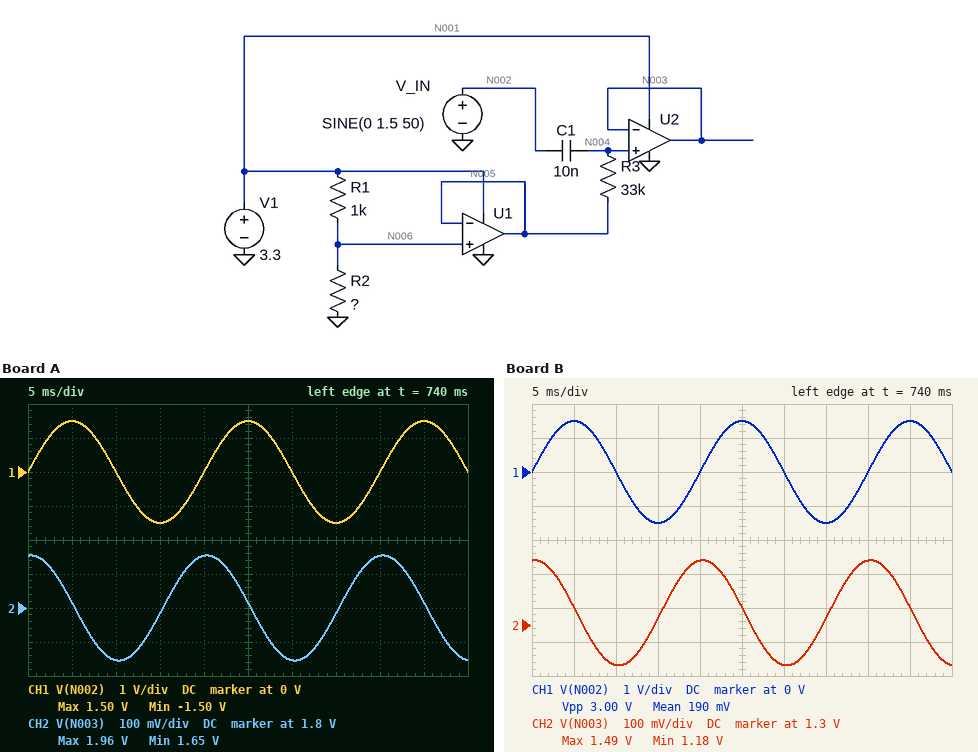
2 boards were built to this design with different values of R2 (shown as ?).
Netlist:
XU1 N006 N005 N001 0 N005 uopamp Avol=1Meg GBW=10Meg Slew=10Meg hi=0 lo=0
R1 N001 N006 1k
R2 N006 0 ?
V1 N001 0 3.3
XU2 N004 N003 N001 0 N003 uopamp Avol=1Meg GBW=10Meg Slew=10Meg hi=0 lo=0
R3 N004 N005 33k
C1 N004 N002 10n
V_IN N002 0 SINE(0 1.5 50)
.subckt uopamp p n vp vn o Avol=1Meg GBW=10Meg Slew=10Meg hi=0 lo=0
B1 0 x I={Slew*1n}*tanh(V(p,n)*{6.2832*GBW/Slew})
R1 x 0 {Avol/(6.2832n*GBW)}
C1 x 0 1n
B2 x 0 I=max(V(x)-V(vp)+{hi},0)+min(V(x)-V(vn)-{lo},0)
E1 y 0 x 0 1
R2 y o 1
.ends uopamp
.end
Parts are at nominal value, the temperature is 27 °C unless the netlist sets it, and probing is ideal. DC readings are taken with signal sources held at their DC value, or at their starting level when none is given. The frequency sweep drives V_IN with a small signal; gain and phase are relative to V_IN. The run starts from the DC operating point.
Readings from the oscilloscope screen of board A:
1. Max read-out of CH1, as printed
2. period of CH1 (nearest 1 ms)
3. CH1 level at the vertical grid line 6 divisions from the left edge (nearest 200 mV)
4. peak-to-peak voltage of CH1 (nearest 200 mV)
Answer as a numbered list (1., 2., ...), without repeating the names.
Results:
1. 1.50 V
2. 20 ms
3. 0 V
4. 3.0 V
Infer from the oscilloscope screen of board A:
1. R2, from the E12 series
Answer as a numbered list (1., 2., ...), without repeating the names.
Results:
1. 1.2 kΩ
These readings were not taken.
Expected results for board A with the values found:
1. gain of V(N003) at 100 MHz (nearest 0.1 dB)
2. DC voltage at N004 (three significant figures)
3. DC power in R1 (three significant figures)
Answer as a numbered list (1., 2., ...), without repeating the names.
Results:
1. -20.0 dB
2. 1.80 V
3. 2.25 mW
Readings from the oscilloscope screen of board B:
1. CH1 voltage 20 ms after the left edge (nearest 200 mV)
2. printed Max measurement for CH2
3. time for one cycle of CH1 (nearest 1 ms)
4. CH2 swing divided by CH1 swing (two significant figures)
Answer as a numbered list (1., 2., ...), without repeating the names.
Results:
1. 0 V
2. 1.49 V
3. 20 ms
4. 0.10
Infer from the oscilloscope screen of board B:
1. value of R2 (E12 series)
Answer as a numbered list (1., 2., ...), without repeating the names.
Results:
1. 680 Ω
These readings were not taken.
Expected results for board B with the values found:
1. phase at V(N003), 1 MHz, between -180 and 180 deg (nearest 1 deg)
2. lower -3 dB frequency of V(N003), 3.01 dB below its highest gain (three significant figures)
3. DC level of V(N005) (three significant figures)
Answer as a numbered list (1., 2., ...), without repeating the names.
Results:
1. -6 deg
2. 482 Hz
3. 1.34 V
